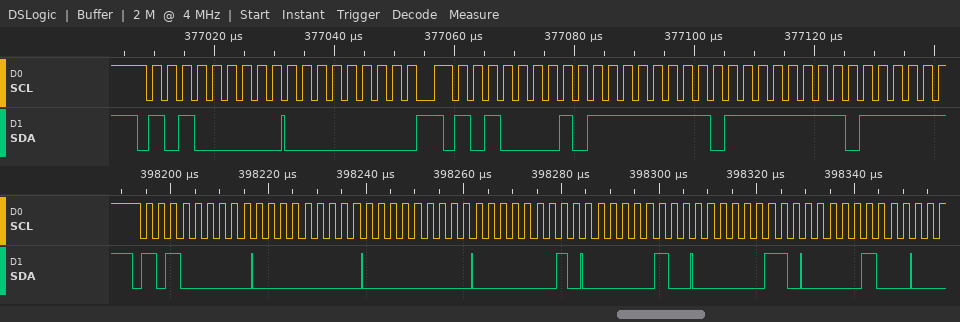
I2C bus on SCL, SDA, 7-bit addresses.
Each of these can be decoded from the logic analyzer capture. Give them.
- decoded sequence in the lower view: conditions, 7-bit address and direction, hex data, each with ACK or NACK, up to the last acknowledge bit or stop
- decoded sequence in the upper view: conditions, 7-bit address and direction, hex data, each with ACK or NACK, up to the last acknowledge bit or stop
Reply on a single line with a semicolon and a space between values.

start, address 50 write ACK, 00 ACK, 00 ACK, 01 ACK, 02 ACK, 03 ACK, 04 ACK; start, address 50 write ACK, 00 ACK, repeated start, address 50 read ACK, FF ACK, FF ACK
